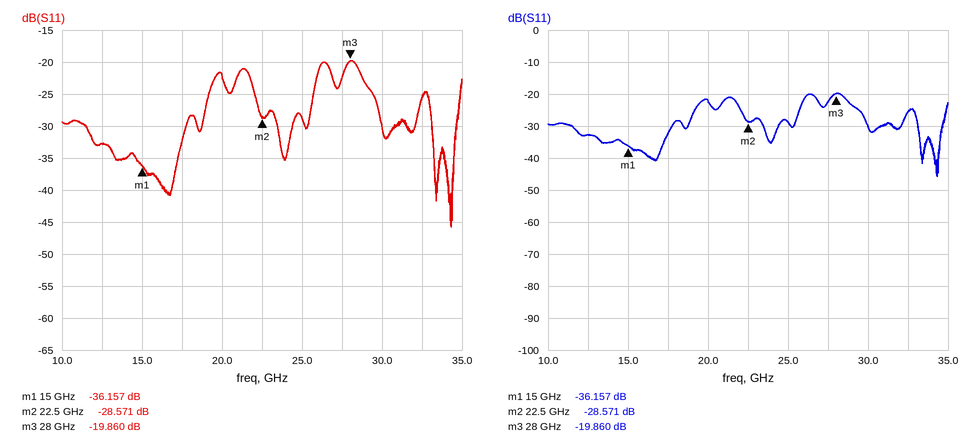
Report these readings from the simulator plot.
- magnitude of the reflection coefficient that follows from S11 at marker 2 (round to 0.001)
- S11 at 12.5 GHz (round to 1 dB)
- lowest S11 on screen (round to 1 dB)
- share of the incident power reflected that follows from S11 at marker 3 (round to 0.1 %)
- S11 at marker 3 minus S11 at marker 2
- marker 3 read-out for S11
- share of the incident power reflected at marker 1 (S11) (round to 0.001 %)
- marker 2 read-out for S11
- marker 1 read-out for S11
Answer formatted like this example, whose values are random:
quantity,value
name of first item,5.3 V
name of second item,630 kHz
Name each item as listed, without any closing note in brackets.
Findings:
quantity,value
magnitude of the reflection coefficient that follows from S11 at marker 2,0.037
S11 at 12.5 GHz,-33 dB
lowest S11 on screen,-46 dB
share of the incident power reflected that follows from S11 at marker 3,1.0 %
S11 at marker 3 minus S11 at marker 2,8.711 dB
marker 3 read-out for S11,-19.860 dB
share of the incident power reflected at marker 1 (S11),0.024 %
marker 2 read-out for S11,-28.571 dB
marker 1 read-out for S11,-36.157 dB
